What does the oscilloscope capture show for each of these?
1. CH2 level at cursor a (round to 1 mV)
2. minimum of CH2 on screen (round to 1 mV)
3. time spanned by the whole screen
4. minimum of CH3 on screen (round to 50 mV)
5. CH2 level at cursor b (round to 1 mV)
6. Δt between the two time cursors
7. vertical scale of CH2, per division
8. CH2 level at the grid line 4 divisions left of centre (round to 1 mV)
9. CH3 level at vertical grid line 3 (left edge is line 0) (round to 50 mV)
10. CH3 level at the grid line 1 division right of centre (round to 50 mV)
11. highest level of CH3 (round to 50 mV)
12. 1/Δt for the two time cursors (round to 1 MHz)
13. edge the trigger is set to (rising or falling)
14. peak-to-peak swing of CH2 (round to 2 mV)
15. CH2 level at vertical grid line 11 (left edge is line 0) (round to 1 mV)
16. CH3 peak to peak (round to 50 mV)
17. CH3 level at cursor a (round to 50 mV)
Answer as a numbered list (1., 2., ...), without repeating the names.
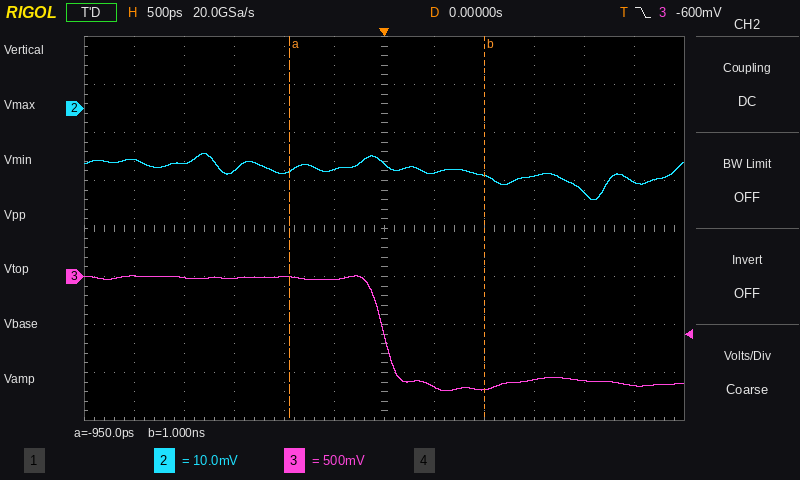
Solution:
1. -13 mV
2. -19 mV
3. 6 ns
4. -1.20 V
5. -14 mV
6. 1.95 ns
7. 10 mV
8. -11 mV
9. 0 mV
10. -1.15 V
11. 0 mV
12. 513 MHz
13. falling
14. 10 mV
15. -15 mV
16. 1.20 V
17. 0 mV
